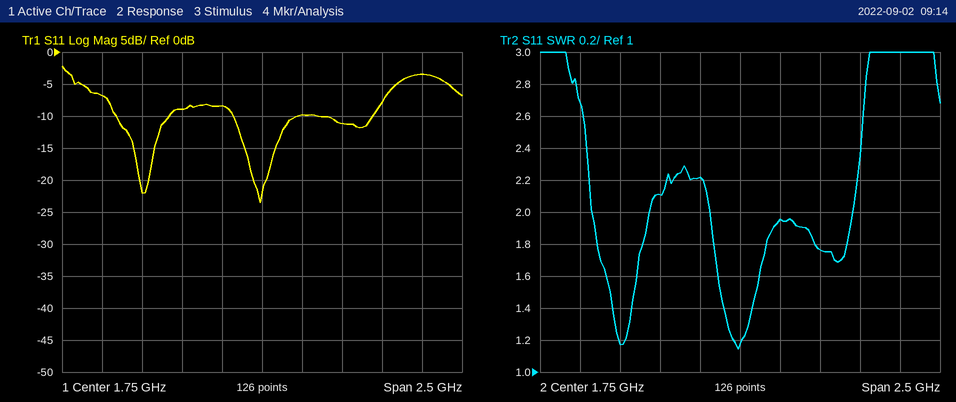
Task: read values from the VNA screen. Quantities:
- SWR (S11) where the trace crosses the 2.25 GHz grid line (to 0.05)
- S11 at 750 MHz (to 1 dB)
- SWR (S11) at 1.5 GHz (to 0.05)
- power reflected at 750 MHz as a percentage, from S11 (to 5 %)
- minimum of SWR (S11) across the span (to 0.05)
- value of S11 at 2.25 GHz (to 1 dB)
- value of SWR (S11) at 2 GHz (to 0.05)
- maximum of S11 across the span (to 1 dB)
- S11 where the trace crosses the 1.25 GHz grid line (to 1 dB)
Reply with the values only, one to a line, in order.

1.75
-7 dB
2.20
20 %
1.15
-11 dB
1.95
-2 dB
-9 dB
